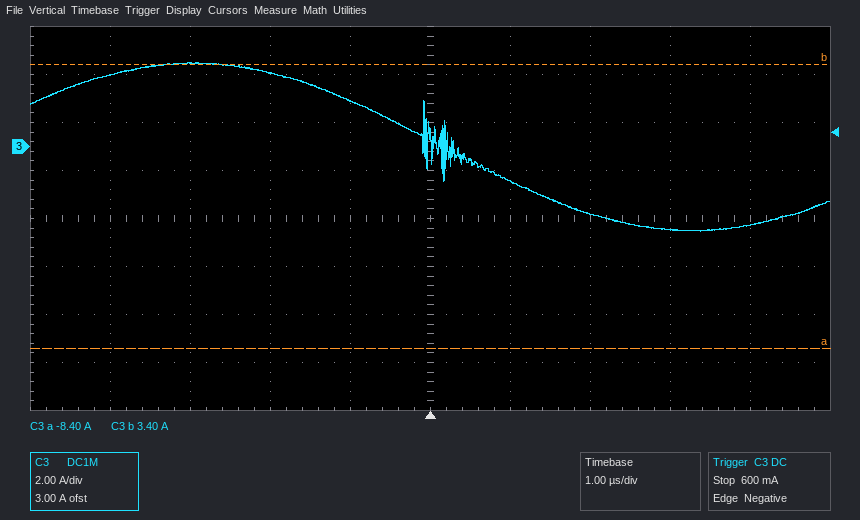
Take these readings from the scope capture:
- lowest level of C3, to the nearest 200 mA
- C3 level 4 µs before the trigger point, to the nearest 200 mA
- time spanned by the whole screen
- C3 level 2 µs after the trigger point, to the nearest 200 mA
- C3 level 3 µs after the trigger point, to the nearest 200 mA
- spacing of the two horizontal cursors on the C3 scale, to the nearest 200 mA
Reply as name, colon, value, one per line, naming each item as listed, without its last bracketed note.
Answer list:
lowest level of C3, to the nearest 200 mA: -3.6 A
C3 level 4 µs before the trigger point, to the nearest 200 mA: 3.0 A
time spanned by the whole screen: 10 µs
C3 level 2 µs after the trigger point, to the nearest 200 mA: -2.8 A
C3 level 3 µs after the trigger point, to the nearest 200 mA: -3.4 A
spacing of the two horizontal cursors on the C3 scale, to the nearest 200 mA: 11.8 A
